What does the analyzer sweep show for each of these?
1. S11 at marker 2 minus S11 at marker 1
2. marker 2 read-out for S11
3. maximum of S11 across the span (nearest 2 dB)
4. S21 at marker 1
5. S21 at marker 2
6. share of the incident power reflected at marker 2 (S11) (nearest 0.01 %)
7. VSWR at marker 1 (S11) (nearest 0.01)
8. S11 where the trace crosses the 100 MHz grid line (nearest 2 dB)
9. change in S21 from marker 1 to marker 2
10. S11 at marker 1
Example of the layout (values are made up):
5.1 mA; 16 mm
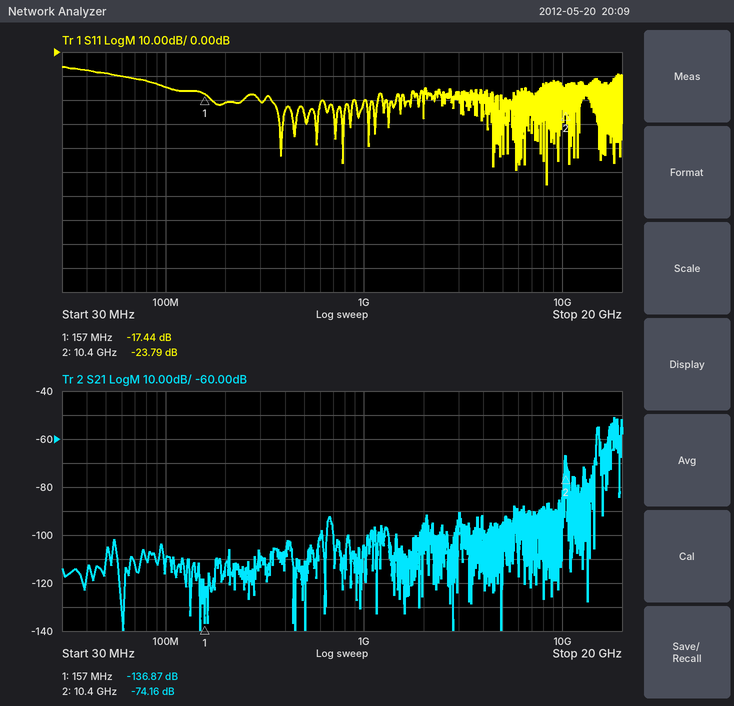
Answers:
-6.35 dB; -23.79 dB; -6 dB; -136.87 dB; -74.16 dB; 0.42 %; 1.31; -14 dB; 62.71 dB; -17.44 dB
